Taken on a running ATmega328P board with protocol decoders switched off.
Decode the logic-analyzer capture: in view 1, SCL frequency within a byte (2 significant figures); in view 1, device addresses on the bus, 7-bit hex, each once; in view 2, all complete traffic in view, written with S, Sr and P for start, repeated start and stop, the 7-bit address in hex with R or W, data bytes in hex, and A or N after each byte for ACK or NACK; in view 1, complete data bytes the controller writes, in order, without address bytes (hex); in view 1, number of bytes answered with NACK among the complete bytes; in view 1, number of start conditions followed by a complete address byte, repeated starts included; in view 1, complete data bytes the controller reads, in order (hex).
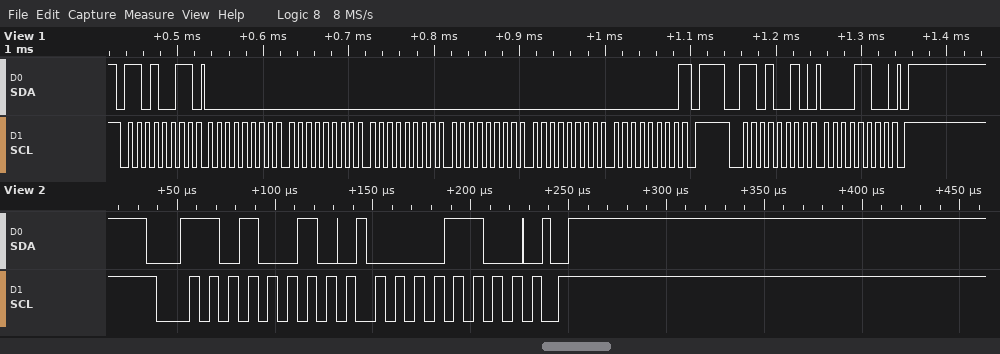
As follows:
100 kHz
0x69
S 69W A 0C A P
0C
1
2
00 00 00 00 00 00
